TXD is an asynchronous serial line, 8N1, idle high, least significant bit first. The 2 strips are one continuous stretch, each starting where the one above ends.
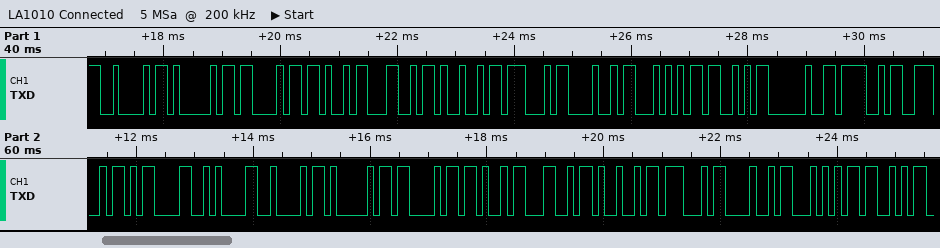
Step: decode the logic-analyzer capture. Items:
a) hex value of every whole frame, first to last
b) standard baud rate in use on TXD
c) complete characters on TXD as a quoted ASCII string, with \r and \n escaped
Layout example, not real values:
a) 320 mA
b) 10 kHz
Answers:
a) 42 41 43 4B 4C 49 47 48 54 53 20 4F 4E 0D 0A 42 41 43 4B 4C 49 47 48 54 53
b) 9600 baud
c) "BACKLIGHTS ON\r\nBACKLIGHTS"
